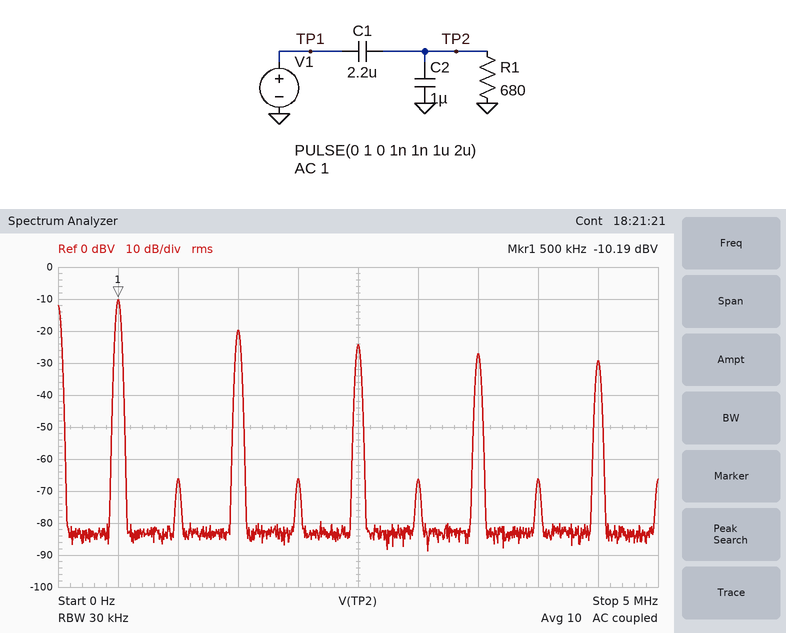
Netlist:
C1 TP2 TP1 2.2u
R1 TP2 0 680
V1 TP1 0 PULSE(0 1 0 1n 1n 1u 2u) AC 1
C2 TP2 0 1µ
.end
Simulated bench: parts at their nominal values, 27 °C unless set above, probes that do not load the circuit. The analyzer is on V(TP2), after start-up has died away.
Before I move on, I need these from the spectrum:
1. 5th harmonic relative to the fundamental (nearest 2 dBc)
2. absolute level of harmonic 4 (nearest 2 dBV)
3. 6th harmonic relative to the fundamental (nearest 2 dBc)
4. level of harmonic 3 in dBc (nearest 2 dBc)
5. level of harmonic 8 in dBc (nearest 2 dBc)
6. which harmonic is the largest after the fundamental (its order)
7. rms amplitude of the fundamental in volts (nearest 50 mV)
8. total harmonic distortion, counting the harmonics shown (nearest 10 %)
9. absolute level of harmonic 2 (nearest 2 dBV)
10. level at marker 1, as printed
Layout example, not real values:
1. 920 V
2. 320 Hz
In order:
1. -14 dBc
2. -66 dBV
3. -56 dBc
4. -10 dBc
5. -56 dBc
6. 3
7. 300 mV
8. 40 %
9. -66 dBV
10. -10.19 dBV
